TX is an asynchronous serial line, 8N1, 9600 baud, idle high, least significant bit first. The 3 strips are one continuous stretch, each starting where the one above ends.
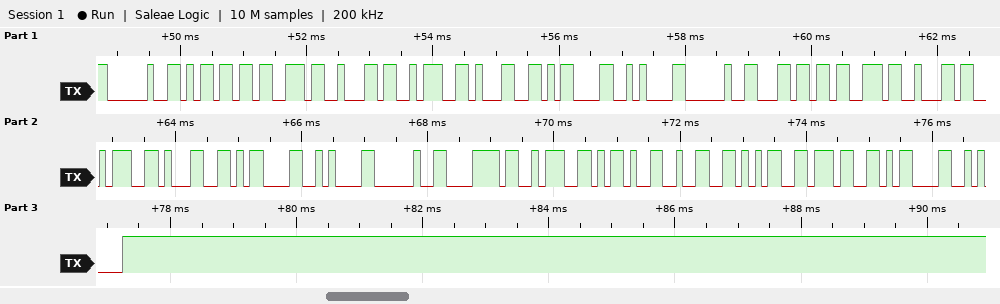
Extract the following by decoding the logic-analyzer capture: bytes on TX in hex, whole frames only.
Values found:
20 6D 73 62 3A 31 0D 0A 20 6C 73 62 3A 31 0D 0A 20 78 3A 2D 32 35 37 0D 0A
